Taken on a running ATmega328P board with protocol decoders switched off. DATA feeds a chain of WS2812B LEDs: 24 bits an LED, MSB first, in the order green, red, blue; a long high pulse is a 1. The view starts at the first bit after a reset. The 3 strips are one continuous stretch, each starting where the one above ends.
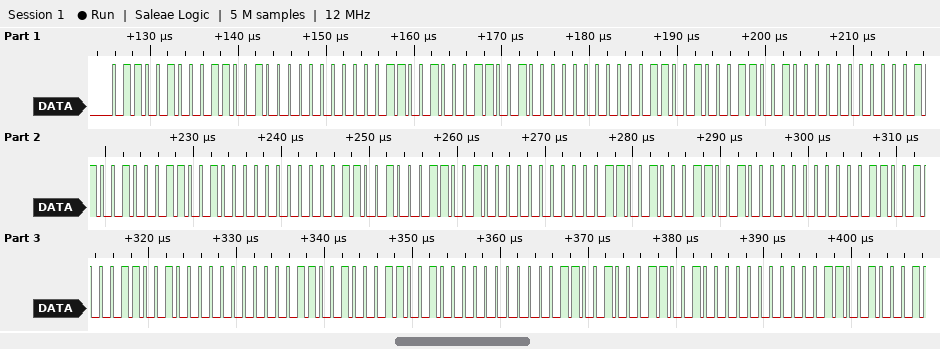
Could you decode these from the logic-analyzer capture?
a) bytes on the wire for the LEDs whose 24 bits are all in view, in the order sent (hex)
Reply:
64 64 00 64 64 00 64 64 00 64 64 00 64 64 00 64 64 00 64 64 00 64 64 00 64 64 00
